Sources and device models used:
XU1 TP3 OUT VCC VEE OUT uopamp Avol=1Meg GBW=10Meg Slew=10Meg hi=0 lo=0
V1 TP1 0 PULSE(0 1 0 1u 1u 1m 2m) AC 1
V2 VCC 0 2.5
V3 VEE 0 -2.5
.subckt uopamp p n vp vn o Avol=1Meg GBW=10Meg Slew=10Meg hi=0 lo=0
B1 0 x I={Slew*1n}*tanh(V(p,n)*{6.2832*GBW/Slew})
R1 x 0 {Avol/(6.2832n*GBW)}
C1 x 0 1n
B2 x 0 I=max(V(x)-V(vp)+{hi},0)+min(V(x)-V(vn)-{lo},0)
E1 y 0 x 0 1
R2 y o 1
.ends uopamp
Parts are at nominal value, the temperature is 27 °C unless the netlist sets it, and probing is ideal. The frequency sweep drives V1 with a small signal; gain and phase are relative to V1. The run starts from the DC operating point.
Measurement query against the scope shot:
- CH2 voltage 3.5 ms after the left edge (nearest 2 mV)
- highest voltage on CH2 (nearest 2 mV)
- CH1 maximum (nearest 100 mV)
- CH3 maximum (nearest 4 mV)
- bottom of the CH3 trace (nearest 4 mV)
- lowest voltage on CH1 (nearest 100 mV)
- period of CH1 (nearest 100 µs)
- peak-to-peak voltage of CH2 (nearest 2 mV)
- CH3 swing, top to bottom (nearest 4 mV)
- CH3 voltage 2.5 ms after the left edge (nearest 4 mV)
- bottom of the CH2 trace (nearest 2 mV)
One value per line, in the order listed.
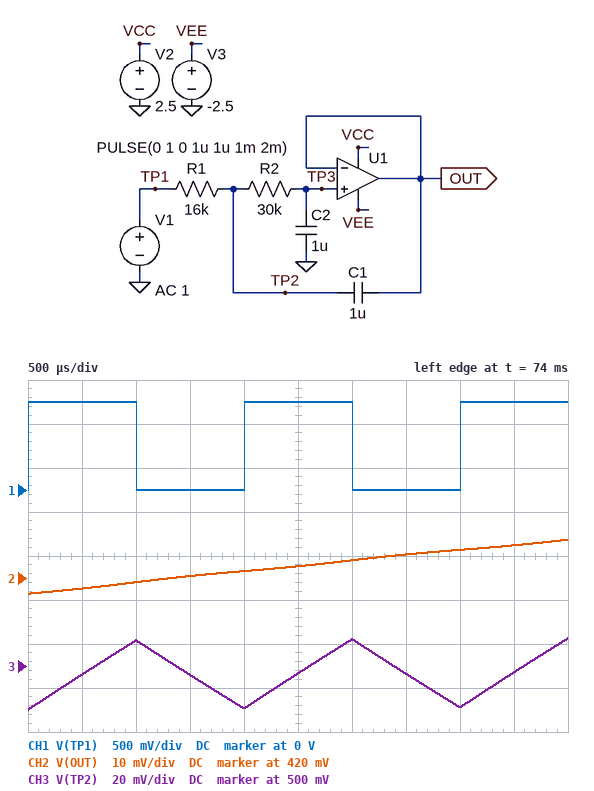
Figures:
426 mV
428 mV
1.0 V
512 mV
480 mV
0 V
2.0 ms
12 mV
32 mV
496 mV
416 mV
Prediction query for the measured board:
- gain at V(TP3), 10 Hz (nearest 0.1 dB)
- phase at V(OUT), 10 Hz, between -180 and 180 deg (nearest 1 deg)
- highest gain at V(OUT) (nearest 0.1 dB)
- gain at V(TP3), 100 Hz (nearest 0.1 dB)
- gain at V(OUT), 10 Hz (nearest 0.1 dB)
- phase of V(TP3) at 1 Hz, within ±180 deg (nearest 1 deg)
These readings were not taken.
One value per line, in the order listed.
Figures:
-9.6 dB
-107 deg
0 dB
-45.6 dB
-9.6 dB
-16 deg
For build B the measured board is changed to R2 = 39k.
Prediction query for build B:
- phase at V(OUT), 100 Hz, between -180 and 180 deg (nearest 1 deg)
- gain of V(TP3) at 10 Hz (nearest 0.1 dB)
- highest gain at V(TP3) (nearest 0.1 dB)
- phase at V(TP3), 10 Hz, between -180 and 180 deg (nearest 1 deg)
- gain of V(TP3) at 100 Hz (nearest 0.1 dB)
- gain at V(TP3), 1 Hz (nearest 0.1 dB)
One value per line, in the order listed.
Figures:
-172 deg
-11.5 dB
0 dB
-113 deg
-47.9 dB
-0.3 dB
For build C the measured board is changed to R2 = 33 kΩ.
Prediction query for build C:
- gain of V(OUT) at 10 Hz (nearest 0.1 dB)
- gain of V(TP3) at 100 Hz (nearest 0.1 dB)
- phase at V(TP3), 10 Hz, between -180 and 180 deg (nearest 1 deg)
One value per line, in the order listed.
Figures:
-10.3 dB
-46.4 dB
-109 deg
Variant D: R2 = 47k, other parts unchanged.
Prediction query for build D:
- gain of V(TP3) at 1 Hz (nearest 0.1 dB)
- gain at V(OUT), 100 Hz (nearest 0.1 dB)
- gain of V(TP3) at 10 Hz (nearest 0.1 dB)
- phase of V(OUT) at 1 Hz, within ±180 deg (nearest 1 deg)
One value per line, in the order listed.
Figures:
-0.4 dB
-49.5 dB
-12.9 dB
-22 deg
